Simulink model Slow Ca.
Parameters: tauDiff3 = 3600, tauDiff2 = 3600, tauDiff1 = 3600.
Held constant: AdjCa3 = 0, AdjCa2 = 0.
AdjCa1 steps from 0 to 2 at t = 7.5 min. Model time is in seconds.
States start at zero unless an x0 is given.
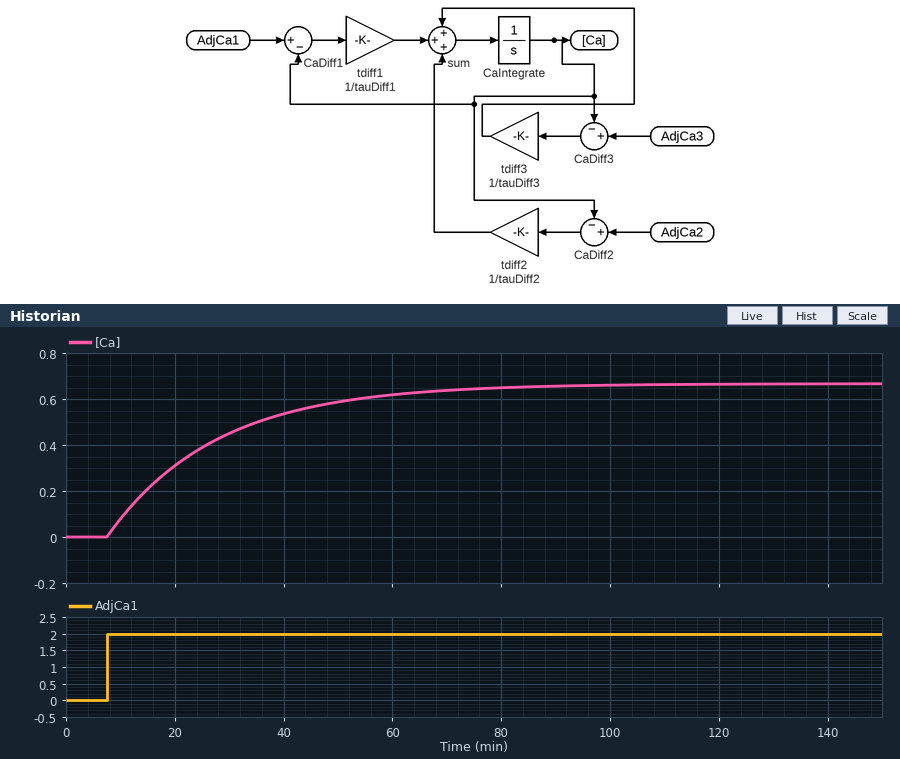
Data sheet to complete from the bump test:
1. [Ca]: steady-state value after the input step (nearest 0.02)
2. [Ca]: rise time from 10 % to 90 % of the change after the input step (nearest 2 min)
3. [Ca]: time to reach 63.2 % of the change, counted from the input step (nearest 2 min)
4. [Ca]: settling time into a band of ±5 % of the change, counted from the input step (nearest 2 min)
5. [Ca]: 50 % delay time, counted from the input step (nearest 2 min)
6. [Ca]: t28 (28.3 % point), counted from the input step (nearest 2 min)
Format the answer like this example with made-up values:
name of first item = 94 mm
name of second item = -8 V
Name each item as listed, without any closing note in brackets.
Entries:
[Ca]: steady-state value after the input step = 0.66
[Ca]: rise time from 10 % to 90 % of the change after the input step = 44 min
[Ca]: time to reach 63.2 % of the change, counted from the input step = 20 min
[Ca]: settling time into a band of ±5 % of the change, counted from the input step = 60 min
[Ca]: 50 % delay time, counted from the input step = 14 min
[Ca]: t28 (28.3 % point), counted from the input step = 6 min
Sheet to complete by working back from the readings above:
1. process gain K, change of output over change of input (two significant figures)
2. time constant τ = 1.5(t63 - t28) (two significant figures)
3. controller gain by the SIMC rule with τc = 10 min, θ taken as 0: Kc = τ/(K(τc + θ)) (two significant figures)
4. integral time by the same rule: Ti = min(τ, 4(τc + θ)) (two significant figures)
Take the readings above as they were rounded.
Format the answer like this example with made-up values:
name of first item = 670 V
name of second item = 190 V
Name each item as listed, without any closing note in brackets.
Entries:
process gain K, change of output over change of input = 0.33
time constant τ = 1.5(t63 - t28) = 21 min
controller gain by the SIMC rule with τc = 10 min, θ taken as 0: Kc = τ/(K(τc + θ)) = 6.4
integral time by the same rule: Ti = min(τ, 4(τc + θ)) = 21 min
